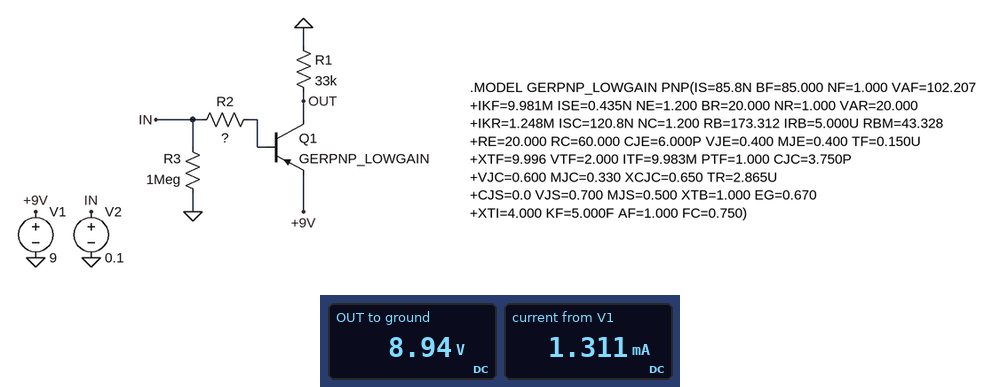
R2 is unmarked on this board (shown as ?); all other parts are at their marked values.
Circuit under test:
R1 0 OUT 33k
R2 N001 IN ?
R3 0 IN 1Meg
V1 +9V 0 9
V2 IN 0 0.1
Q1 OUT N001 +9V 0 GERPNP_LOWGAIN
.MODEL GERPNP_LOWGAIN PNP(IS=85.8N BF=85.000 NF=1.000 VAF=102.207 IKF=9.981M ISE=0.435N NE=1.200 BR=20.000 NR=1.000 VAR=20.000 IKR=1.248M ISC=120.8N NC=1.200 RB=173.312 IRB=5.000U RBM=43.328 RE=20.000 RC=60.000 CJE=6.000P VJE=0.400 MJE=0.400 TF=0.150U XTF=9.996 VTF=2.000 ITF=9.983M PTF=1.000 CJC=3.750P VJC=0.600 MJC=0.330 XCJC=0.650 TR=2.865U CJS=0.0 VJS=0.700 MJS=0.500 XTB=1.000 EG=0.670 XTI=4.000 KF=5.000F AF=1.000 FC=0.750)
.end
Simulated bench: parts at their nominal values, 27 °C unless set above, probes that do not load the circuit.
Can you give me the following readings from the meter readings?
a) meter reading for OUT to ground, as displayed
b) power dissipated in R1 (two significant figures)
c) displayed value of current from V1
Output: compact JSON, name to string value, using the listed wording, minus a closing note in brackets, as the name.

{"meter reading for OUT to ground, as displayed": "8.94 V", "power dissipated in R1": "2.4 mW", "displayed value of current from V1": "1.311 mA"}
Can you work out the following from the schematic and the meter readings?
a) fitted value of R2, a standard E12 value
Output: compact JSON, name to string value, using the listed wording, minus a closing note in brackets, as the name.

{"fitted value of R2, a standard E12 value": "8.2 kΩ"}
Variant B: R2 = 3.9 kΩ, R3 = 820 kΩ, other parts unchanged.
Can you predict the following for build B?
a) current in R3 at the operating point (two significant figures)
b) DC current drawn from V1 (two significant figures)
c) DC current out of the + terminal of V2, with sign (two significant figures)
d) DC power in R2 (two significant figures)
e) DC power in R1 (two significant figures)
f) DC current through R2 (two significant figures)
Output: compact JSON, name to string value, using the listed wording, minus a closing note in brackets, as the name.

{"current in R3 at the operating point": "120 nA", "DC current drawn from V1": "2.4 mA", "DC current out of the + terminal of V2, with sign": "-2.2 mA", "DC power in R2": "18 mW", "DC power in R1": "2.4 mW", "DC current through R2": "2.2 mA"}
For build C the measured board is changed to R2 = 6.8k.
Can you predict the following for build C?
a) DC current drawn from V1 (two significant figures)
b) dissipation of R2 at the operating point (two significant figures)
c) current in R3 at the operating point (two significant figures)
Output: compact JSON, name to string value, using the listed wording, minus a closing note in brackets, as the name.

{"DC current drawn from V1": "1.5 mA", "dissipation of R2 at the operating point": "11 mW", "current in R3 at the operating point": "100 nA"}
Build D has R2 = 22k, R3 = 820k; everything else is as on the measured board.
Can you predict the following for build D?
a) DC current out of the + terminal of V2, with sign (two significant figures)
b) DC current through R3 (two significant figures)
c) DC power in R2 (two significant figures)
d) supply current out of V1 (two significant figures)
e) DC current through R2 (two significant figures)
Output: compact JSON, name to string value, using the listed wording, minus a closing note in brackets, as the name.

{"DC current out of the + terminal of V2, with sign": "-390 µA", "DC current through R3": "120 nA", "DC power in R2": "3.4 mW", "supply current out of V1": "660 µA", "DC current through R2": "390 µA"}
